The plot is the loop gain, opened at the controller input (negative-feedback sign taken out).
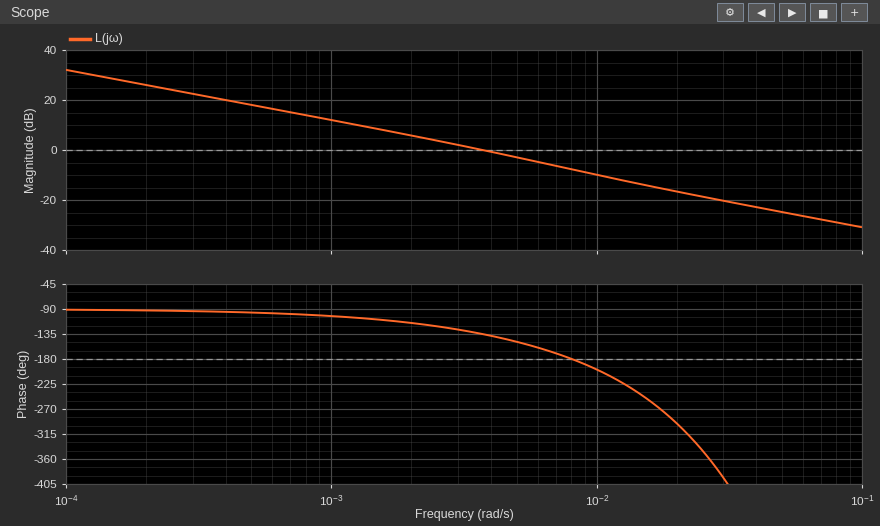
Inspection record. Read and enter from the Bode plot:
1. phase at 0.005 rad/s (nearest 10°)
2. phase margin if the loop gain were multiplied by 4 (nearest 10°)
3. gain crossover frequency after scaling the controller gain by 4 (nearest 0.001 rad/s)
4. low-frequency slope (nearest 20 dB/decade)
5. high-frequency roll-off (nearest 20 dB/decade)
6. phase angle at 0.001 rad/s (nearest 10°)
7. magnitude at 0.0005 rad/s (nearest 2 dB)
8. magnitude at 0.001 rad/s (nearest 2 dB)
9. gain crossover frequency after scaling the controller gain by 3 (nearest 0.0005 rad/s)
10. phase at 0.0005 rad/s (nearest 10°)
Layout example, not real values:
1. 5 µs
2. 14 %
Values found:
1. -150°
2. -40°
3. 0.012 rad/s
4. -20 dB/decade
5. -20 dB/decade
6. -100°
7. 18 dB
8. 12 dB
9. 0.0095 rad/s
10. -100°
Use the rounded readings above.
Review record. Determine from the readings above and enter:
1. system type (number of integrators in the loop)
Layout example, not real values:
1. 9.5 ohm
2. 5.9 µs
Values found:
1. 1
